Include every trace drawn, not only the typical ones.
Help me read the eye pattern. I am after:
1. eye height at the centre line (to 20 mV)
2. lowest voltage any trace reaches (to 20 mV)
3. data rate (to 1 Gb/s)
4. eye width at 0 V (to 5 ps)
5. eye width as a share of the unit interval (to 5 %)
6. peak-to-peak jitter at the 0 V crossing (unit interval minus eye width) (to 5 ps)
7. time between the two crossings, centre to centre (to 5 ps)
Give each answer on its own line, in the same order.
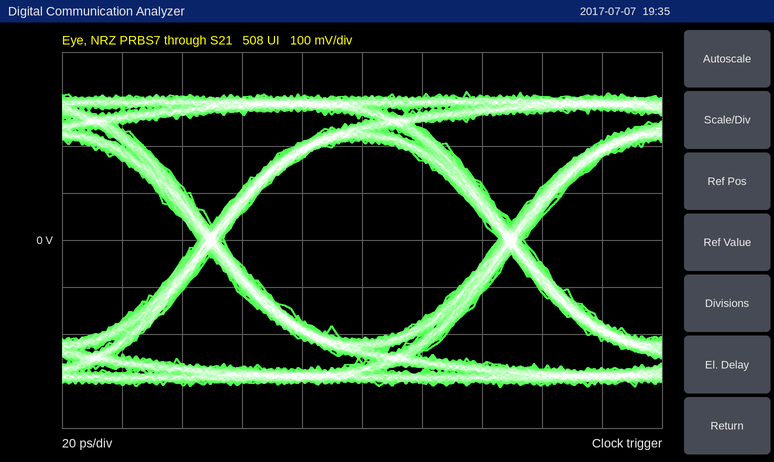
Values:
420 mV
-320 mV
10 Gb/s
90 ps
90 %
10 ps
100 ps
